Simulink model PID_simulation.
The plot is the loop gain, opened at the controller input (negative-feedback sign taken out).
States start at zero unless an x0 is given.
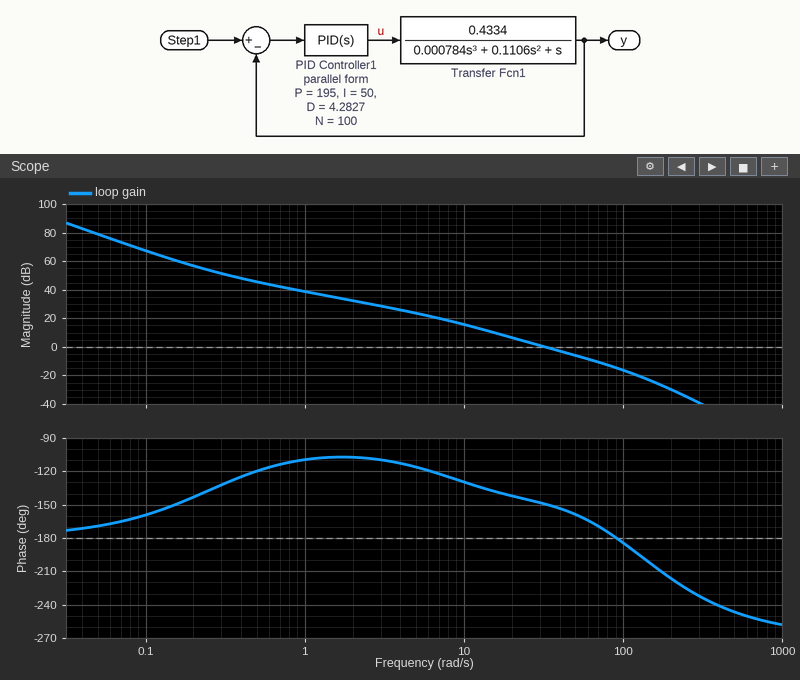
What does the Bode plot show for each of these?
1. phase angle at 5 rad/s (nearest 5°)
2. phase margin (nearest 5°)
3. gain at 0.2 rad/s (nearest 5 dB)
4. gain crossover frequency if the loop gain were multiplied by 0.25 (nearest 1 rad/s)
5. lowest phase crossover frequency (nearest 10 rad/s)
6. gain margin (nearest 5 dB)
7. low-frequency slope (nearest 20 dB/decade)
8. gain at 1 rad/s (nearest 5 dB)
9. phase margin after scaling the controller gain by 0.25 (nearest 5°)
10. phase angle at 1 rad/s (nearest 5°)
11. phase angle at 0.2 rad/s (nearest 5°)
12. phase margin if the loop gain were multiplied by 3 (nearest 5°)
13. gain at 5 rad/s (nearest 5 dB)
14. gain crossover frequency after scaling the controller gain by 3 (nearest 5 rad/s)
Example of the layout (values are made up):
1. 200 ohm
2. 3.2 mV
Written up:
1. -115°
2. 30°
3. 55 dB
4. 13 rad/s
5. 90 rad/s
6. 15 dB
7. -40 dB/decade
8. 40 dB
9. 45°
10. -110°
11. -145°
12. 15°
13. 25 dB
14. 65 rad/s
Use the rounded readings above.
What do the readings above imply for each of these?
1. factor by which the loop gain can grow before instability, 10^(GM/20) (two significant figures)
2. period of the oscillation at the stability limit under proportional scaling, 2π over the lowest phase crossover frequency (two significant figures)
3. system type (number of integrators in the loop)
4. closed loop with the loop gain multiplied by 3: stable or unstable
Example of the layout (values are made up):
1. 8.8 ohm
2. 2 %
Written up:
1. 5.6
2. 0.070 s
3. 2
4. stable
